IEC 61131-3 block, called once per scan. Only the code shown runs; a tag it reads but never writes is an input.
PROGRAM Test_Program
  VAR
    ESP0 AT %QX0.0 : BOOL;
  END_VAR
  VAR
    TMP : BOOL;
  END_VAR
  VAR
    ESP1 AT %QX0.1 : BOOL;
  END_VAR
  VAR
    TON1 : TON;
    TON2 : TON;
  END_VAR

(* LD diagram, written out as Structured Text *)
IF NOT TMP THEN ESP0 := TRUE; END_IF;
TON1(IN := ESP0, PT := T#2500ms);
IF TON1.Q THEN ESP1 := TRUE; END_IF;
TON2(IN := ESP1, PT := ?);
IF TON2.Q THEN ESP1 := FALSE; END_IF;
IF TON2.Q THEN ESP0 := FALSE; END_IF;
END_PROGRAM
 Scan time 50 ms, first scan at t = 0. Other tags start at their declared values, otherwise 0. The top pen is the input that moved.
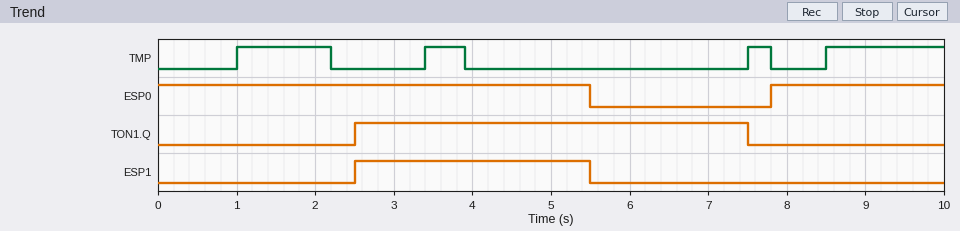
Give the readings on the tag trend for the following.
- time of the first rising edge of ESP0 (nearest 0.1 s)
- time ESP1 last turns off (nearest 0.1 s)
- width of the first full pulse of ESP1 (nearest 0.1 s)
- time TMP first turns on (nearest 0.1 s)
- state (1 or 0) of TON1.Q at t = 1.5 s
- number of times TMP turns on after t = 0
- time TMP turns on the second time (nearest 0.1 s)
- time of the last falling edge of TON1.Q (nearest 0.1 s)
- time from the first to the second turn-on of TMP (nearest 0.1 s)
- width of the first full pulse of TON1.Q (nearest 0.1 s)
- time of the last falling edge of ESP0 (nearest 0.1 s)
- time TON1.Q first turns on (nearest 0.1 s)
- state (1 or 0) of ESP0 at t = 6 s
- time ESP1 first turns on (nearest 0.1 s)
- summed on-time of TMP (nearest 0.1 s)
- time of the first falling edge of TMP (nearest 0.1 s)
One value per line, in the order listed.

7.8 s
5.5 s
3.0 s
1.0 s
0
4
3.4 s
7.5 s
2.4 s
5.0 s
5.5 s
2.5 s
0
2.5 s
3.5 s
2.2 s
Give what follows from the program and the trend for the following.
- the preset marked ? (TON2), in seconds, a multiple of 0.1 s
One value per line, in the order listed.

3.0 s
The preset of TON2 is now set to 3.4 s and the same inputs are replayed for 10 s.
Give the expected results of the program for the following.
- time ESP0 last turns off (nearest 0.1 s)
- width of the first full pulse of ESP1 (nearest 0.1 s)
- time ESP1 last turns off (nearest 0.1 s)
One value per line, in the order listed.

5.9 s
3.4 s
5.9 s
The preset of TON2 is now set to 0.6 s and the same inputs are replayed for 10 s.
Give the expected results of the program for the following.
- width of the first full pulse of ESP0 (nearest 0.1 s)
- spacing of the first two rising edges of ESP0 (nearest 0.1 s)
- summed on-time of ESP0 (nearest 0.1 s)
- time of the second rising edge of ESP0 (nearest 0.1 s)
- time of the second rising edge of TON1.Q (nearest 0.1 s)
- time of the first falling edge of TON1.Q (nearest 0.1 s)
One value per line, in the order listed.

3.1 s
3.9 s
8.4 s
7.8 s
6.4 s
3.4 s
